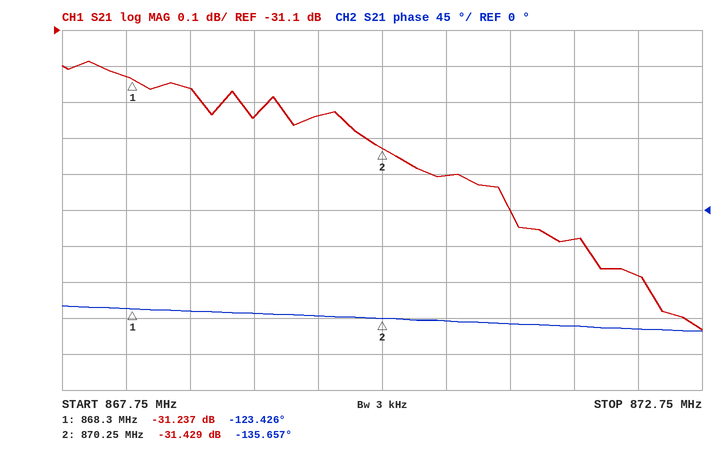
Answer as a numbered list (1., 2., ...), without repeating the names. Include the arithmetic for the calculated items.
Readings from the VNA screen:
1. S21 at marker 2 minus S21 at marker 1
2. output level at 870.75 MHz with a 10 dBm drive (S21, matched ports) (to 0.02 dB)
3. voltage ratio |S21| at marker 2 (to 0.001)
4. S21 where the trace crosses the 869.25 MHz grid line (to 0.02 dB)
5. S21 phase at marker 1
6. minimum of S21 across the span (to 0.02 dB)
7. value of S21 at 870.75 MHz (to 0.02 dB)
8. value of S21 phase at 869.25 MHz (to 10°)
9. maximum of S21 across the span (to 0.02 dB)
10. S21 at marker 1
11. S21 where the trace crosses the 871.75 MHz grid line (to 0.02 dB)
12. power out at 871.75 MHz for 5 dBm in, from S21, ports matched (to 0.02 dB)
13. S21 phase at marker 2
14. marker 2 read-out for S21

1. -31.429 − (-31.237) = -0.192 dB
2. 10 dBm + (-31.50 dB) = -21.50 dBm
3. 10^(-31.429/20) ≈ 0.027
4. -31.34 dB
5. -123.426°
6. -31.94 dB
7. -31.50 dB
8. -130°
9. -31.18 dB
10. -31.237 dB
11. -31.68 dB
12. 5 dBm + (-31.68 dB) = -26.68 dBm
13. -135.657°
14. -31.429 dB
